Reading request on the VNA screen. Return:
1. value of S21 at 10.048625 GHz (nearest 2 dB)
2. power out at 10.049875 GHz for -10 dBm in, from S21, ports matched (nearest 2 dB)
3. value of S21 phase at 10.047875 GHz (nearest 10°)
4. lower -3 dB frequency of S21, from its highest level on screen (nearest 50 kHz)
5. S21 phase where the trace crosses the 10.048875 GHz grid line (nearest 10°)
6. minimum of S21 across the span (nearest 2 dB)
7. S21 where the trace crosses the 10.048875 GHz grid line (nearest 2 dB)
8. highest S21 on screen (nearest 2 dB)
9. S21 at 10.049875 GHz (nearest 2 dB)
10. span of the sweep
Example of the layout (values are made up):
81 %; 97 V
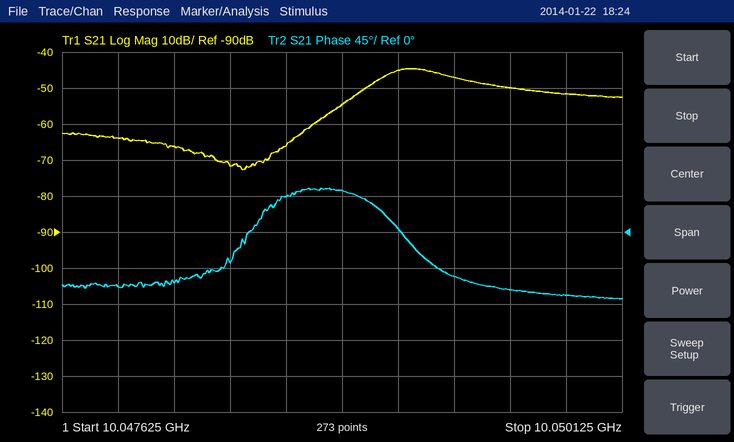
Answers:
-66 dB; -62 dBm; -70°; 10.04905 GHz; 50°; -72 dB; -54 dB; -44 dB; -52 dB; 2.5 MHz
